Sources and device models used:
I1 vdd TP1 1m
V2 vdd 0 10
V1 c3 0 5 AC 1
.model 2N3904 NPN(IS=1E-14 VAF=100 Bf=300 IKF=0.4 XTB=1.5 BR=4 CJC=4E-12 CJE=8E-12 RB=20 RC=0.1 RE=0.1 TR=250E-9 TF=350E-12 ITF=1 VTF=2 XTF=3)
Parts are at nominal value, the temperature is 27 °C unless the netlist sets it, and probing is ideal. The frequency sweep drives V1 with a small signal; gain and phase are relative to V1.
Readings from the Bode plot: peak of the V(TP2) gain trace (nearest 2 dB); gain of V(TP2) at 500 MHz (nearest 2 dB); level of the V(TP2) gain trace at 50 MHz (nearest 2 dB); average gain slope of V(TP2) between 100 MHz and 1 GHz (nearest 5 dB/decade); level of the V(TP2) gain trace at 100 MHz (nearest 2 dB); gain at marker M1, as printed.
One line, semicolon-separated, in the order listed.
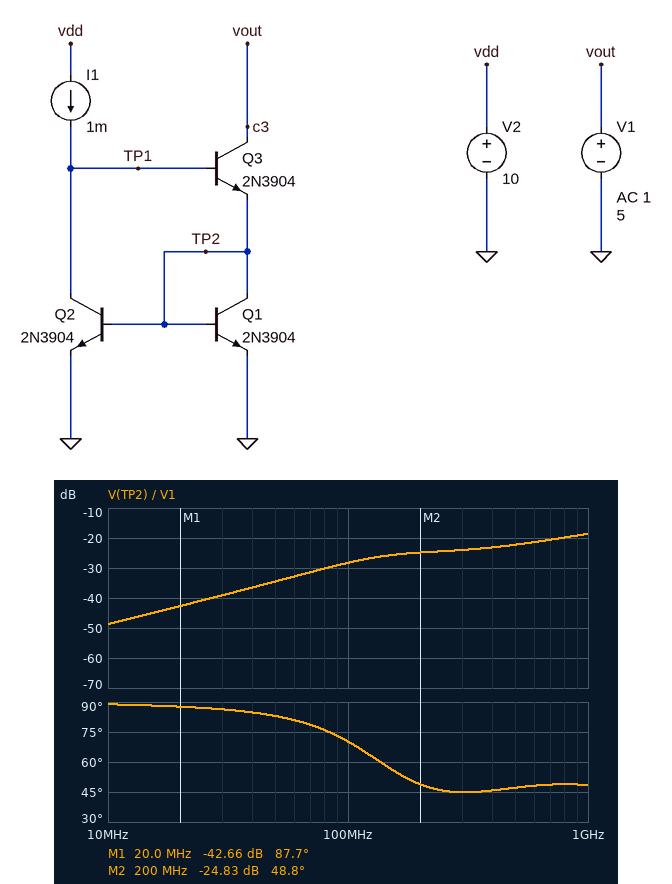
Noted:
-18 dB; -22 dB; -34 dB; 10 dB/decade; -28 dB; -42.66 dB
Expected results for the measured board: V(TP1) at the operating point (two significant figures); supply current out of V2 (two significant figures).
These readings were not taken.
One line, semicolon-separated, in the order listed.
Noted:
1.3 V; 1.0 mA
